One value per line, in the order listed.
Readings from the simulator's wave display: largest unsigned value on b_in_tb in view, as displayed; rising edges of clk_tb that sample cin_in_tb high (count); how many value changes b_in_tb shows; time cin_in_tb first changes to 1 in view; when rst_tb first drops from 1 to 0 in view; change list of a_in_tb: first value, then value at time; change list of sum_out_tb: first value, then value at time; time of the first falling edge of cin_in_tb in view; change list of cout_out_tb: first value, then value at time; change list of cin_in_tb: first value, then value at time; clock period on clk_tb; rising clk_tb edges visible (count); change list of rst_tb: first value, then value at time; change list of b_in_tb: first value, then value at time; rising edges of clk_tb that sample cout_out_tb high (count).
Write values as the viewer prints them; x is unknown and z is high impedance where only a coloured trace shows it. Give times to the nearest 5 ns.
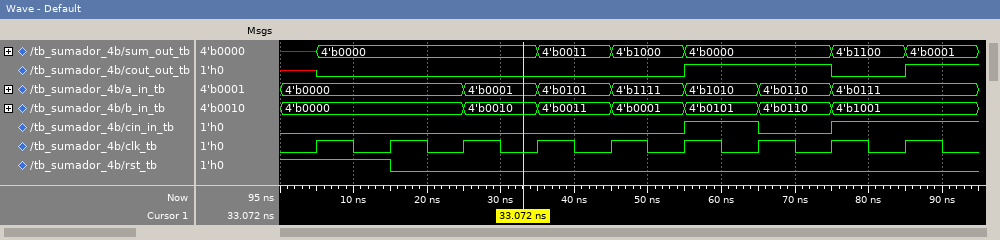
4'b1001
2
6
55 ns
15 ns
4'b0000, 4'b0001 at 25 ns, 4'b0101 at 35 ns, 4'b1111 at 45 ns, 4'b1010 at 55 ns, 4'b0110 at 65 ns, 4'b0111 at 75 ns
x, 4'b0000 at 5 ns, 4'b0011 at 35 ns, 4'b1000 at 45 ns, 4'b0000 at 55 ns, 4'b1100 at 75 ns, 4'b0001 at 85 ns
65 ns
x, 0 at 5 ns, 1 at 55 ns, 0 at 75 ns, 1 at 85 ns
0, 1 at 55 ns, 0 at 65 ns, 1 at 75 ns
10 ns
9
1, 0 at 15 ns
4'b0000, 4'b0010 at 25 ns, 4'b0011 at 35 ns, 4'b0001 at 45 ns, 4'b0101 at 55 ns, 4'b0110 at 65 ns, 4'b1001 at 75 ns
2
